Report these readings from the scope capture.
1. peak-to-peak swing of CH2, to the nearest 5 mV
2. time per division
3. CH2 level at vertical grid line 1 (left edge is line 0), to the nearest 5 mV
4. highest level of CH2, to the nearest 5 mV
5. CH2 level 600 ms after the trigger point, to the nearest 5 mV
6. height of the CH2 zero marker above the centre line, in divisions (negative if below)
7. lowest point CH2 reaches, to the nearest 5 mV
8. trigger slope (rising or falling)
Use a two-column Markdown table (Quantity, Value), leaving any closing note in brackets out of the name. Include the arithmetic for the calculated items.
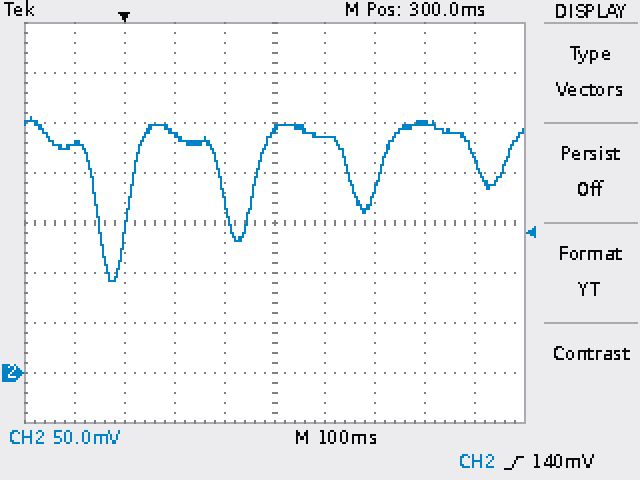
| Quantity | Value |
|---|---|
| peak-to-peak swing of CH2, to the nearest 5 mV | 255 mV − (90 mV) = 165 mV |
| time per division | 100 ms |
| CH2 level at vertical grid line 1 (left edge is line 0), to the nearest 5 mV | 230 mV |
| highest level of CH2, to the nearest 5 mV | 255 mV |
| CH2 level 600 ms after the trigger point, to the nearest 5 mV | 250 mV |
| height of the CH2 zero marker above the centre line, in divisions | -3.0 div |
| lowest point CH2 reaches, to the nearest 5 mV | 90 mV |
| trigger slope | rising |
